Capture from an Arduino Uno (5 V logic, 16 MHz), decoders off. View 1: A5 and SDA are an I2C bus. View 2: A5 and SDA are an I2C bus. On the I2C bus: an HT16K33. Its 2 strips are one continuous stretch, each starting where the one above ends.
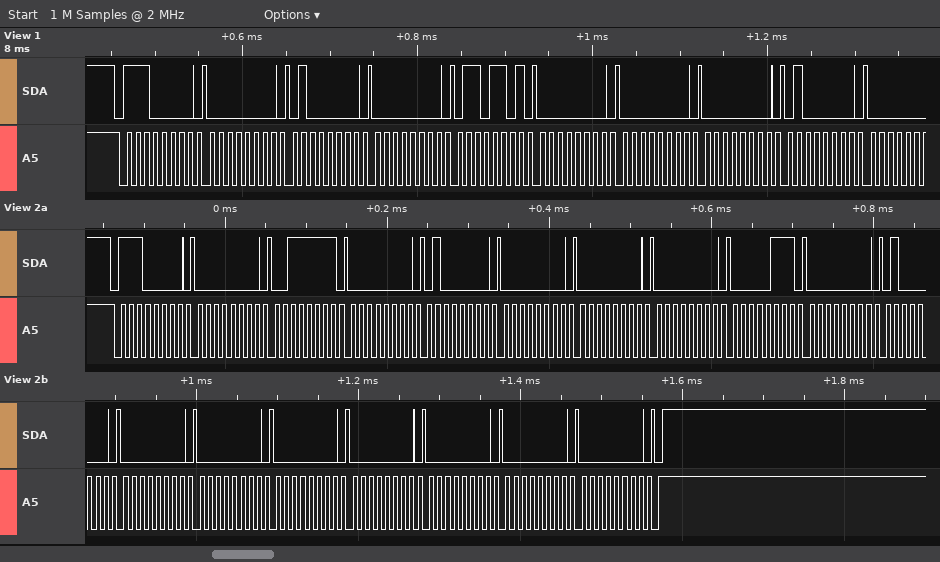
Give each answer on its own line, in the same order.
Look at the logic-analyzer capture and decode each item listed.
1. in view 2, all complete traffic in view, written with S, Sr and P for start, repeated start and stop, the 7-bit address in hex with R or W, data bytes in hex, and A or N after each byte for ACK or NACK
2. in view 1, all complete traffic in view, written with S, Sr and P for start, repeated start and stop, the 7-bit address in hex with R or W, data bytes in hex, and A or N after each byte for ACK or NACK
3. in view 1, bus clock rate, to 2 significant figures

S 70W A 00 A 3F A 00 A 40 A 00 A 00 A 00 A 07 A 00 A 40 A 00 A 00 A 00 A 00 A 00 A 00 A 00 A P
S 70W A 00 A 40 A 00 A 6D A 00 A 00 A 00 A 40 A
100 kHz
